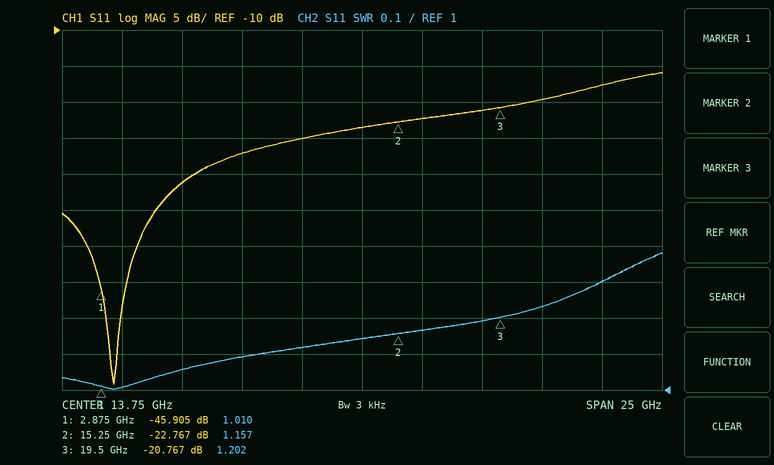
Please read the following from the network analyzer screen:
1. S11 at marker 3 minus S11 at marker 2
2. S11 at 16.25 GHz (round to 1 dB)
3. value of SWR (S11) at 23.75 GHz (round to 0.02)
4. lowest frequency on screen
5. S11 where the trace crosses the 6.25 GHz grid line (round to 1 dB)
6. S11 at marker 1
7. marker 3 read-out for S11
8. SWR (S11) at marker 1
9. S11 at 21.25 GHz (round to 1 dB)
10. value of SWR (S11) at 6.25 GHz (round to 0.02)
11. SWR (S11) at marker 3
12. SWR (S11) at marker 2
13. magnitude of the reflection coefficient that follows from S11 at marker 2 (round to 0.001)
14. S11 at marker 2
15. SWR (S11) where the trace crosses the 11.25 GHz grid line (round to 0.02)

2.000 dB
-22 dB
1.30
1.25 GHz
-31 dB
-45.905 dB
-20.767 dB
1.010
-20 dB
1.06
1.202
1.157
0.073
-22.767 dB
1.12
